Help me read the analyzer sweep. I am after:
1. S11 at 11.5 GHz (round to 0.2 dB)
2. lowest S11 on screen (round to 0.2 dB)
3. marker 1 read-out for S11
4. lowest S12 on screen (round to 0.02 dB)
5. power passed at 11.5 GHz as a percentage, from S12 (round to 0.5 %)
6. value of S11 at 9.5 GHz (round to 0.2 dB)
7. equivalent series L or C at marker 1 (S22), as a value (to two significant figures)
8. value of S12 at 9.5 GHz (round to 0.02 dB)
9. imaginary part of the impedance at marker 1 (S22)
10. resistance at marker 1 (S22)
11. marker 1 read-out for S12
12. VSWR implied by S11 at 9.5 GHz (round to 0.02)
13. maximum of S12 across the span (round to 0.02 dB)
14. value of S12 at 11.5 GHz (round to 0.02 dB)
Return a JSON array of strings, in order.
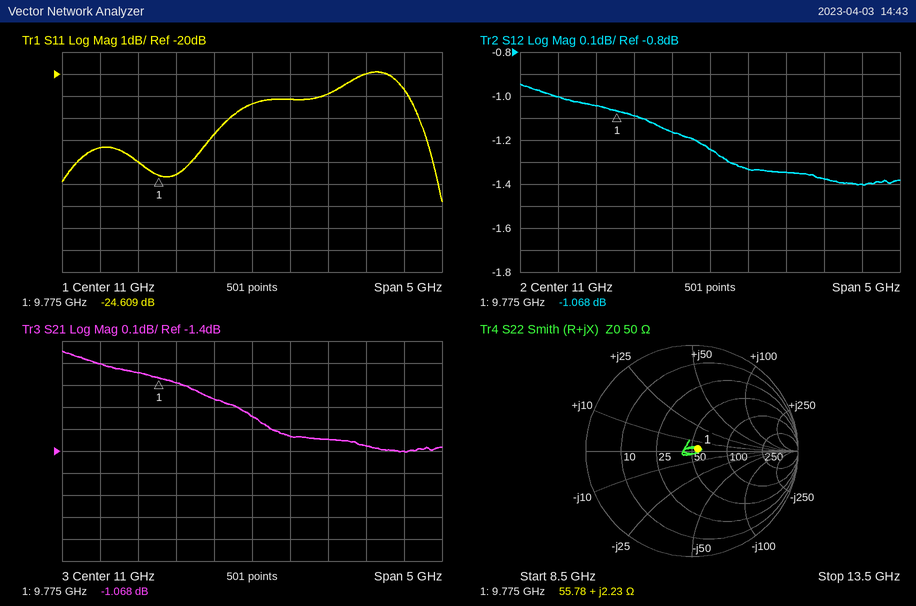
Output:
["-21.2 dB", "-25.8 dB", "-24.609 dB", "-1.40 dB", "73.5 %", "-24.0 dB", "36 pH", "-1.04 dB", "+2.23 Ω", "55.78 Ω", "-1.068 dB", "1.14", "-0.94 dB", "-1.34 dB"]
